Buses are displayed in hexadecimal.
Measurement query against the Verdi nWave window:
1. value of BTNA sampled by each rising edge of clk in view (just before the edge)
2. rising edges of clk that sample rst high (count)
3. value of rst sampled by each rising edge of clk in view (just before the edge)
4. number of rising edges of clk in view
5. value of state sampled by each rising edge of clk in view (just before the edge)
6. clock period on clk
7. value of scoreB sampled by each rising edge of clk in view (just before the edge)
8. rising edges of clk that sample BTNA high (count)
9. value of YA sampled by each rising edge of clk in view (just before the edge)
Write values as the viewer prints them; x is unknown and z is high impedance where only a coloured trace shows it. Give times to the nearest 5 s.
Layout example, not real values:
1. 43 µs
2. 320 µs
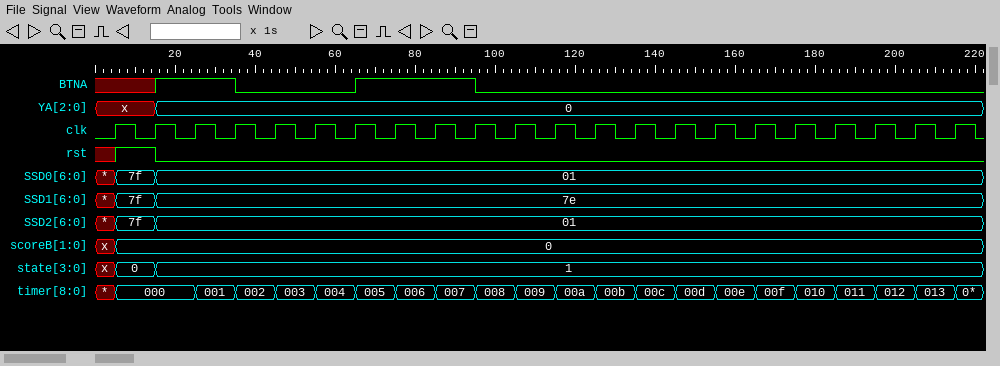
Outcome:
1. x x 1 1 0 0 0 1 1 1 0 0 0 0 0 0 0 0 0 0 0 0
2. 1
3. x 1 0 0 0 0 0 0 0 0 0 0 0 0 0 0 0 0 0 0 0 0
4. 22
5. x, 0, 1, 1, 1, 1, 1, 1, 1, 1, 1, 1, 1, 1, 1, 1, 1, 1, 1, 1, 1, 1
6. 10 s
7. x, 0, 0, 0, 0, 0, 0, 0, 0, 0, 0, 0, 0, 0, 0, 0, 0, 0, 0, 0, 0, 0
8. 5
9. x, x, 0, 0, 0, 0, 0, 0, 0, 0, 0, 0, 0, 0, 0, 0, 0, 0, 0, 0, 0, 0
